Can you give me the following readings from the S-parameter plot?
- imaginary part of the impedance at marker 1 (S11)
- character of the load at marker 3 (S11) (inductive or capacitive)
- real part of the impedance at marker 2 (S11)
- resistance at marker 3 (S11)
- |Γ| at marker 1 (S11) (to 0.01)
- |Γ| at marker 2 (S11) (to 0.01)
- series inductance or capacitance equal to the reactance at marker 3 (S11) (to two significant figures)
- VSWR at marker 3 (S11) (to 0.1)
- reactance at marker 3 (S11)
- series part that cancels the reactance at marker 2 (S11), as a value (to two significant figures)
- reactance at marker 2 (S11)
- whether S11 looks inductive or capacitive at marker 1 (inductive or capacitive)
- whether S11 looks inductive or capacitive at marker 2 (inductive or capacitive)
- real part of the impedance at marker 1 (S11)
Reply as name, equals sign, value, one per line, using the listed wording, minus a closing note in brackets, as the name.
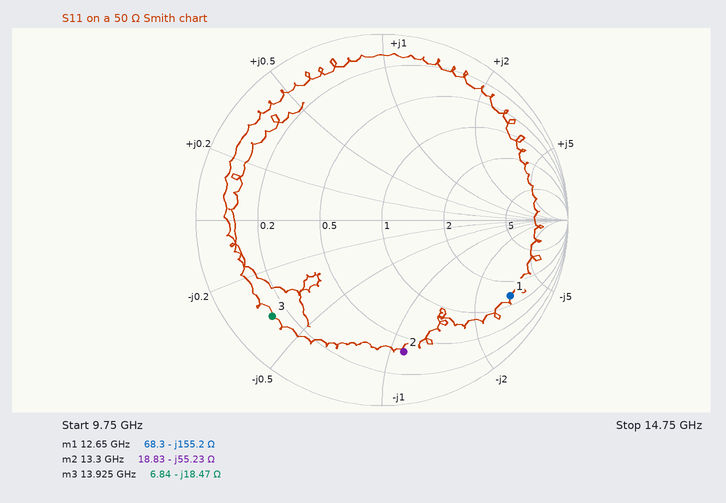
imaginary part of the impedance at marker 1 = -155.2 Ω
character of the load at marker 3 (S11) = capacitive
real part of the impedance at marker 2 = 18.83 Ω
resistance at marker 3 = 6.84 Ω
|Γ| at marker 1 (S11) = 0.80
|Γ| at marker 2 (S11) = 0.72
series inductance or capacitance equal to the reactance at marker 3 (S11) = 620 fF
VSWR at marker 3 (S11) = 8.3
reactance at marker 3 = -18.47 Ω
series part that cancels the reactance at marker 2 (S11), as a value = 660 pH
reactance at marker 2 = -55.23 Ω
whether S11 looks inductive or capacitive at marker 1 = capacitive
whether S11 looks inductive or capacitive at marker 2 = capacitive
real part of the impedance at marker 1 = 68.3 Ω
